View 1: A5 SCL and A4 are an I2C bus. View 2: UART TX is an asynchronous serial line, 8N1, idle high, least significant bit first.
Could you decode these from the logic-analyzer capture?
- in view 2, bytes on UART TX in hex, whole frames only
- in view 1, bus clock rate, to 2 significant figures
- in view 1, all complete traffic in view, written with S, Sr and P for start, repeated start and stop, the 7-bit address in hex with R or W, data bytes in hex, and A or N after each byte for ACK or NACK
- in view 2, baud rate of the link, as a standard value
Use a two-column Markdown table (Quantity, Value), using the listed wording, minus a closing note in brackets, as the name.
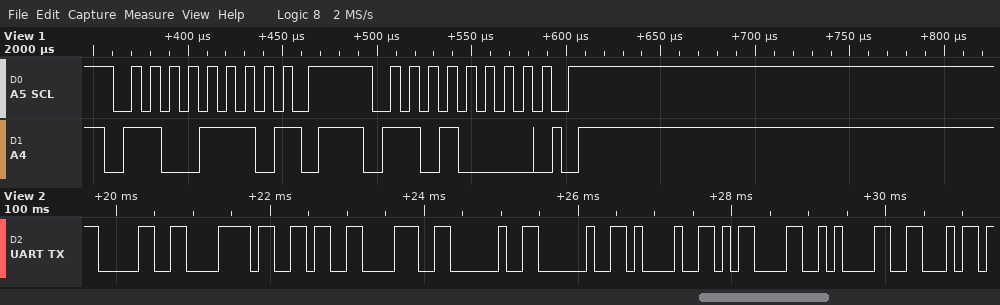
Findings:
| Quantity | Value |
|---|---|
| in view 2, bytes on UART TX in hex, whole frames only | 30 78 36 38 20 20 21 0D 0A 46 |
| in view 1, bus clock rate, to 2 significant figures | 100 kHz |
| in view 1, all complete traffic in view, written with S, Sr and P for start, repeated start and stop, the 7-bit address in hex with R or W, data bytes in hex, and A or N after each byte for ACK or NACK | S 67W N P S 68W A P |
| in view 2, baud rate of the link, as a standard value | 9600 baud |
